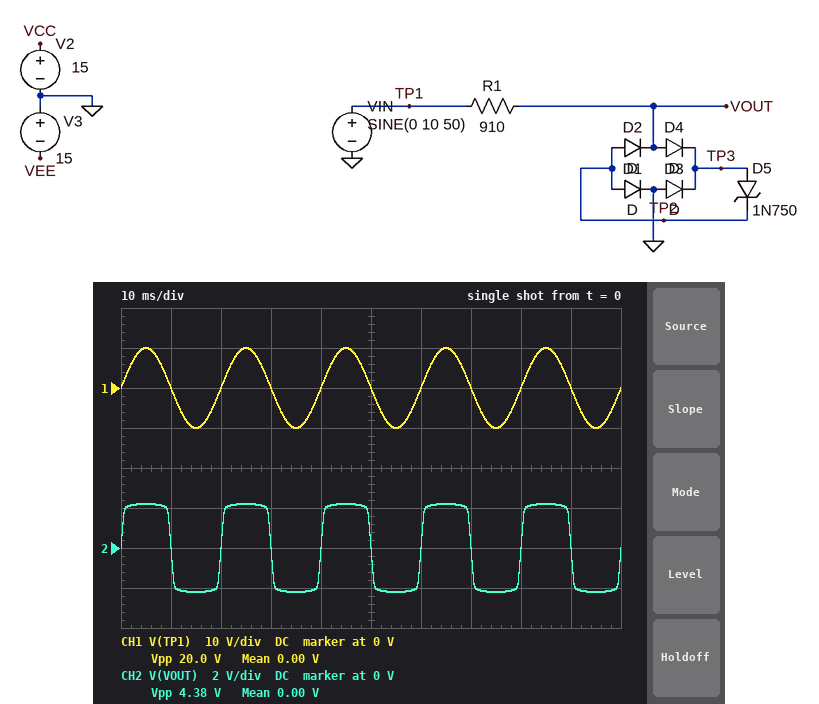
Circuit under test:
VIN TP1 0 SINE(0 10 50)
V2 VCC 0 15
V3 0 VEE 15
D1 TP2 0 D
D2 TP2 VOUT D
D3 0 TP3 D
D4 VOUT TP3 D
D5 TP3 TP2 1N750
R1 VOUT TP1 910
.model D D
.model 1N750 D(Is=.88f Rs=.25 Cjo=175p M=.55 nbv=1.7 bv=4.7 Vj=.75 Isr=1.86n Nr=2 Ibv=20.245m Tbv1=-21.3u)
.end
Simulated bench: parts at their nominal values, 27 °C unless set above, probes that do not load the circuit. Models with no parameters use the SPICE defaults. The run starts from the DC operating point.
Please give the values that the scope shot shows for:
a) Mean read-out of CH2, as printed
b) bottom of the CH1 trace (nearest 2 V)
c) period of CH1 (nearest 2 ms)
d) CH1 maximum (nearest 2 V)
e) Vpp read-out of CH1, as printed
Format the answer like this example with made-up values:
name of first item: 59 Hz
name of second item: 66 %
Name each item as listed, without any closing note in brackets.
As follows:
Mean read-out of CH2, as printed: 0.00 V
bottom of the CH1 trace: -10 V
period of CH1: 20 ms
CH1 maximum: 10 V
Vpp read-out of CH1, as printed: 20.0 V
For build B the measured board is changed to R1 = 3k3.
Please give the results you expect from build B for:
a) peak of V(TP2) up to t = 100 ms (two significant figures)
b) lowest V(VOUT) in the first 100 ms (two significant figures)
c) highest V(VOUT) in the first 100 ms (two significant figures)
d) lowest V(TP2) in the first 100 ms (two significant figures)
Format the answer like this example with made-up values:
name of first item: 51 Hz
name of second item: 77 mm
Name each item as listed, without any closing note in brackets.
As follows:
peak of V(TP2) up to t = 100 ms: 680 mV
lowest V(VOUT) in the first 100 ms: -2.1 V
highest V(VOUT) in the first 100 ms: 2.1 V
lowest V(TP2) in the first 100 ms: -1.4 V
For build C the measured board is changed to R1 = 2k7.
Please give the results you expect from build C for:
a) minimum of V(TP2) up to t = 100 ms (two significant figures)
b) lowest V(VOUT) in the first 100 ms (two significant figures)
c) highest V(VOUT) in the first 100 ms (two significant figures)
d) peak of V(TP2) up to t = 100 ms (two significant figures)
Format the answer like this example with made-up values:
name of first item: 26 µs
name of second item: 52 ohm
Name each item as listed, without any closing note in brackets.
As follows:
minimum of V(TP2) up to t = 100 ms: -1.4 V
lowest V(VOUT) in the first 100 ms: -2.1 V
highest V(VOUT) in the first 100 ms: 2.1 V
peak of V(TP2) up to t = 100 ms: 680 mV
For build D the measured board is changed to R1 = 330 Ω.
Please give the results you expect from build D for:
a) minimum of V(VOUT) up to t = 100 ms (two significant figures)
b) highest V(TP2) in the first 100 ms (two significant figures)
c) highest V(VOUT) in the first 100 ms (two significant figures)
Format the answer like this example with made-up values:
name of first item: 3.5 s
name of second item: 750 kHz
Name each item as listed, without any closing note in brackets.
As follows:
minimum of V(VOUT) up to t = 100 ms: -2.3 V
highest V(TP2) in the first 100 ms: 740 mV
highest V(VOUT) in the first 100 ms: 2.3 V
